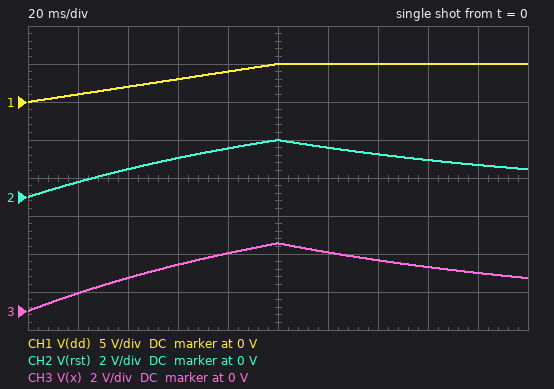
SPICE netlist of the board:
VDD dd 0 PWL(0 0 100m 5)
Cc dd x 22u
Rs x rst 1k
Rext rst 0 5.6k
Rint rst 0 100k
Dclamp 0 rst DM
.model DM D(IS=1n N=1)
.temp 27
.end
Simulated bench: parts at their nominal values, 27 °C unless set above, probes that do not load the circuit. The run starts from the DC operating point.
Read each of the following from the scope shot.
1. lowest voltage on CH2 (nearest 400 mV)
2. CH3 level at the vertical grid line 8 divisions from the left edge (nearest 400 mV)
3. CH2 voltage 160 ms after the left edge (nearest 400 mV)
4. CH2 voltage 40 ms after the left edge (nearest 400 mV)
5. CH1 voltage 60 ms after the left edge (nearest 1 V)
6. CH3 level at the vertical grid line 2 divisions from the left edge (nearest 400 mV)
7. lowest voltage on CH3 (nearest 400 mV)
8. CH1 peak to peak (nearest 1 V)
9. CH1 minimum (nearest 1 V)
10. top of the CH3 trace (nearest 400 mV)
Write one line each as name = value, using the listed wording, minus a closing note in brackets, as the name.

lowest voltage on CH2 = 0 V
CH3 level at the vertical grid line 8 divisions from the left edge = 2.4 V
CH2 voltage 160 ms after the left edge = 2.0 V
CH2 voltage 40 ms after the left edge = 1.6 V
CH1 voltage 60 ms after the left edge = 3 V
CH3 level at the vertical grid line 2 divisions from the left edge = 1.6 V
lowest voltage on CH3 = 0 V
CH1 peak to peak = 5 V
CH1 minimum = 0 V
top of the CH3 trace = 3.6 V
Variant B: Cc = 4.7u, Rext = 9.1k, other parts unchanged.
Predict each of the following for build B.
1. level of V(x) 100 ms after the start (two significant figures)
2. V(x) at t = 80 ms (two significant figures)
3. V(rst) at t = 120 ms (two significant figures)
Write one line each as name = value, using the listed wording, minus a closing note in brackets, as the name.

level of V(x) 100 ms after the start = 2.0 V
V(x) at t = 80 ms = 1.8 V
V(rst) at t = 120 ms = 1.1 V
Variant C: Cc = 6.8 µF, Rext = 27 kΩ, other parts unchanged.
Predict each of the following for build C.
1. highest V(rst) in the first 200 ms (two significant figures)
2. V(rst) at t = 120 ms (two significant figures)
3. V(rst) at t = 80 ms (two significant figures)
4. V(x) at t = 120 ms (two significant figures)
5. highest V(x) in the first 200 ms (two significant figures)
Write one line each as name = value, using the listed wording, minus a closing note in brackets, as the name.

highest V(rst) in the first 200 ms = 3.5 V
V(rst) at t = 120 ms = 3.1 V
V(rst) at t = 80 ms = 3.0 V
V(x) at t = 120 ms = 3.2 V
highest V(x) in the first 200 ms = 3.7 V
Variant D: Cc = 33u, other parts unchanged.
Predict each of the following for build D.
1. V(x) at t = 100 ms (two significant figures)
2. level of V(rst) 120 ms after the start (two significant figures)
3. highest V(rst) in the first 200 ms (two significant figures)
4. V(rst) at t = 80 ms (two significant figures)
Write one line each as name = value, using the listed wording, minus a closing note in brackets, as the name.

V(x) at t = 100 ms = 4.0 V
level of V(rst) 120 ms after the start = 3.0 V
highest V(rst) in the first 200 ms = 3.3 V
V(rst) at t = 80 ms = 2.8 V
